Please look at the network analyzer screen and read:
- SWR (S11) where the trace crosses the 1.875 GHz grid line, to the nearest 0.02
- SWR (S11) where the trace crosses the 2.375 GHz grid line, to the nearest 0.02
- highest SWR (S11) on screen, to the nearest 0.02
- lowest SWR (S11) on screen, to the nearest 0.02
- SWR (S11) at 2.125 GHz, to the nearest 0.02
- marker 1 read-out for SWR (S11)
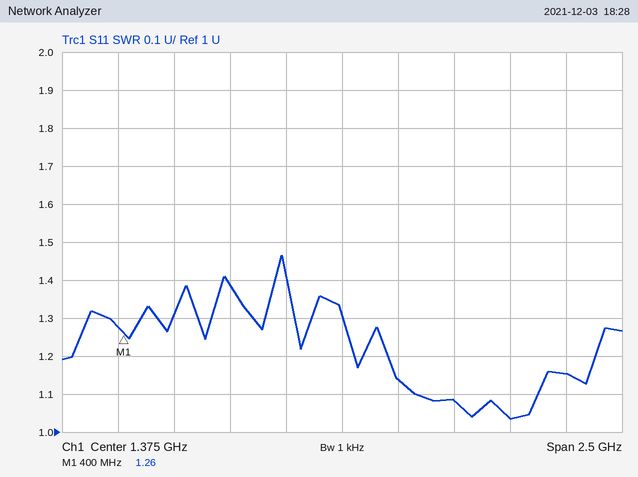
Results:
1.08
1.16
1.46
1.04
1.04
1.26
